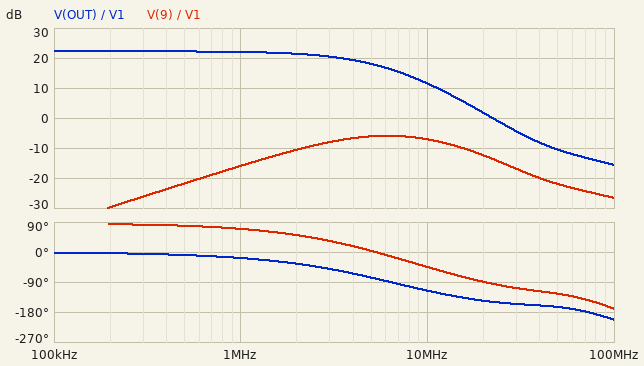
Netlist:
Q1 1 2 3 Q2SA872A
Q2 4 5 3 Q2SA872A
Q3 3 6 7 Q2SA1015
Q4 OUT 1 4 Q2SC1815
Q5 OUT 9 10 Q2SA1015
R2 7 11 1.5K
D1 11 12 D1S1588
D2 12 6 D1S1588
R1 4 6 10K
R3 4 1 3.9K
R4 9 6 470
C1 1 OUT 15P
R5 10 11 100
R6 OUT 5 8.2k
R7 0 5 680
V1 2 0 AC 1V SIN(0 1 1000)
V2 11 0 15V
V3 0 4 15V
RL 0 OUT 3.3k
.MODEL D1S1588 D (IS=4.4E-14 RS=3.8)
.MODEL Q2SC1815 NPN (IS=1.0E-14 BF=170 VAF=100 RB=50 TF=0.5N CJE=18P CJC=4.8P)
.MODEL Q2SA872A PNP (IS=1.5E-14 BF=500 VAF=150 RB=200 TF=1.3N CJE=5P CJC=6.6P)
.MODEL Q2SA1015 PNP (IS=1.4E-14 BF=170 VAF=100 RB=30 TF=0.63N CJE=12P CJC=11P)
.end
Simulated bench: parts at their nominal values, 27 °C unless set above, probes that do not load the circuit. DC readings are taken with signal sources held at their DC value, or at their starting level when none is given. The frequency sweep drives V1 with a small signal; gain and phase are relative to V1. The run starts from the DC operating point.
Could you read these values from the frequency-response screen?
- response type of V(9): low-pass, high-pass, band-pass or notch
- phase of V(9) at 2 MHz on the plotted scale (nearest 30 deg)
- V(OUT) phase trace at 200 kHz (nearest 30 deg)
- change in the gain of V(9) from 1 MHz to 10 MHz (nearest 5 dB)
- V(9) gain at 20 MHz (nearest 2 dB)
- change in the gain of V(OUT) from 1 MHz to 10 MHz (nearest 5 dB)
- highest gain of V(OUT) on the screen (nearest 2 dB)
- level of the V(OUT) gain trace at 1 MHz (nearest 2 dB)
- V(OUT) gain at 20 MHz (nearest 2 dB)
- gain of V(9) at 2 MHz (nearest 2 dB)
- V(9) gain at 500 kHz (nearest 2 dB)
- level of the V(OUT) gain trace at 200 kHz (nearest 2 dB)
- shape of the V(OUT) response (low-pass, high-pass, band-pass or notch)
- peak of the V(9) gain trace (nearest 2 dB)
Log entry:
band-pass
60 deg
0 deg
10 dB
-12 dB
-10 dB
22 dB
22 dB
2 dB
-10 dB
-22 dB
22 dB
low-pass
-6 dB
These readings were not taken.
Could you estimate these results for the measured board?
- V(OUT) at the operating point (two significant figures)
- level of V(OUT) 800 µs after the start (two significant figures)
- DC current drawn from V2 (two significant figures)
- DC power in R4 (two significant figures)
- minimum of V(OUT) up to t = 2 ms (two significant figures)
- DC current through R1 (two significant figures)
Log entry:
-52 mV
-12 V
9.3 mA
450 nW
-13 V
2.9 mA
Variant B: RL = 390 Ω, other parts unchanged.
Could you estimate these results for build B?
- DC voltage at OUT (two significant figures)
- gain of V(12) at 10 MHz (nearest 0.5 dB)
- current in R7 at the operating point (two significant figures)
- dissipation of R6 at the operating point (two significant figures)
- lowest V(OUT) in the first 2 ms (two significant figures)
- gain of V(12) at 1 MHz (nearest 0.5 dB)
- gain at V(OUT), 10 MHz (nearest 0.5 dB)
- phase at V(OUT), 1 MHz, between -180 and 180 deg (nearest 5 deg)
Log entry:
-50 mV
-40.5 dB
5.2 µA
260 nW
-12 V
-47.5 dB
10.5 dB
-20 deg
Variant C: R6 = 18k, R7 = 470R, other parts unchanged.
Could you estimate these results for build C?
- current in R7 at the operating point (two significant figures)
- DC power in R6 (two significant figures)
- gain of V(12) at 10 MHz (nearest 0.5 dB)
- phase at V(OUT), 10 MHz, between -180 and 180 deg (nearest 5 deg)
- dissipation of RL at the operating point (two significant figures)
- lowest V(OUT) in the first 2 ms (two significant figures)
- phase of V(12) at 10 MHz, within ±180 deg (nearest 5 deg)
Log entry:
7.8 µA
1.2 µW
-40.5 dB
-120 deg
6.9 µW
-15 V
-45 deg
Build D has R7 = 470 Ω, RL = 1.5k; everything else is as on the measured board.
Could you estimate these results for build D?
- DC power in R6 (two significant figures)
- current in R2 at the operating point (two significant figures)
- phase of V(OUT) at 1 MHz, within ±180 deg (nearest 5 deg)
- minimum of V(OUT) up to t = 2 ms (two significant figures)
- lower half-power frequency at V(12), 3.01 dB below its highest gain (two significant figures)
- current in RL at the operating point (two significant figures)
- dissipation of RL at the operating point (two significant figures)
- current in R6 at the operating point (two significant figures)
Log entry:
550 nW
460 µA
-25 deg
-15 V
87 MHz
47 µA
3.4 µW
8.2 µA
